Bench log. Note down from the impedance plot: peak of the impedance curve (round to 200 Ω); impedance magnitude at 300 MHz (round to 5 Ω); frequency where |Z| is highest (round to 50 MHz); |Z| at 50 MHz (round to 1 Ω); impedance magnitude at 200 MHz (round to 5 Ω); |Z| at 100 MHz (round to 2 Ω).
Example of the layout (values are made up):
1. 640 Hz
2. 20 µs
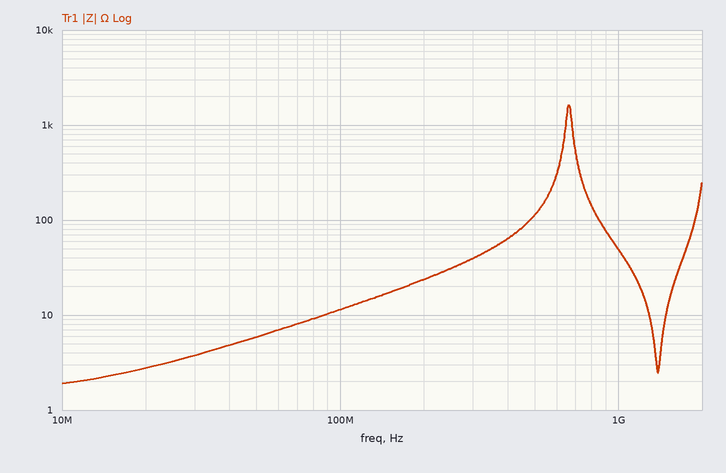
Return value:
1. 1.6 kΩ
2. 40 Ω
3. 650 MHz
4. 6 Ω
5. 25 Ω
6. 12 Ω
